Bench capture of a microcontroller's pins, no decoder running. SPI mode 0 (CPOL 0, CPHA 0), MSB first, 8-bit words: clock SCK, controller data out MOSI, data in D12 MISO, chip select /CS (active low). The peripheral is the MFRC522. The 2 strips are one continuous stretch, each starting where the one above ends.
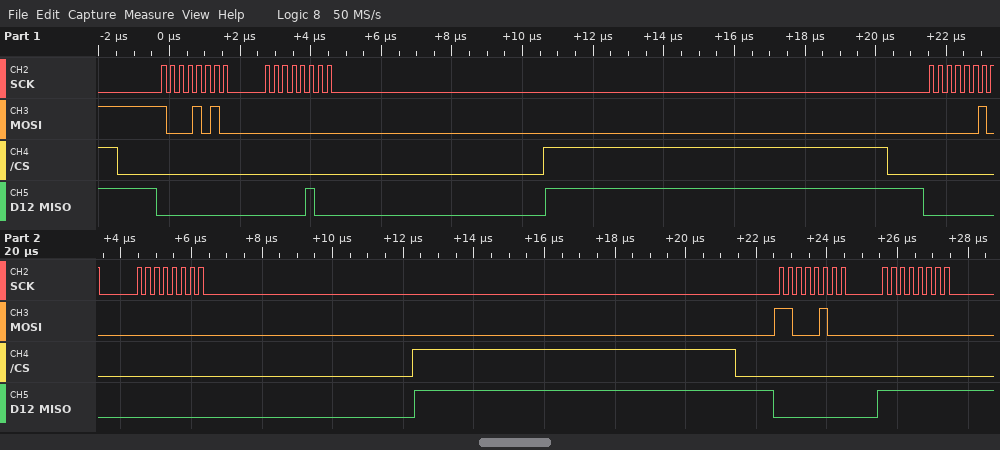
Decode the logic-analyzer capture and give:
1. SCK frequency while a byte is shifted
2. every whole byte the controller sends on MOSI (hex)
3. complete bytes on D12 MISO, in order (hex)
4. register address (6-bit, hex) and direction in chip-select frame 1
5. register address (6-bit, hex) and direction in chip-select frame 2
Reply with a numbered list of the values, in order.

1. 4 MHz
2. 0x8A 0x00 0x02 0x00 0xC4 0x00
3. 0x00 0x04 0x00 0x00 0x00 0xFF
4. 0x05 read
5. 0x01 write
